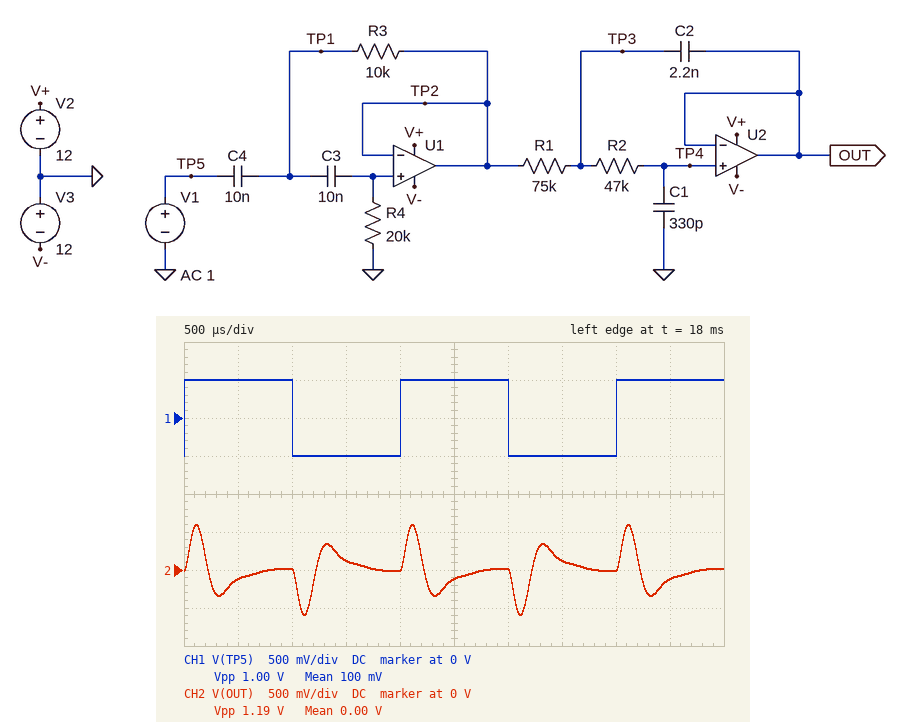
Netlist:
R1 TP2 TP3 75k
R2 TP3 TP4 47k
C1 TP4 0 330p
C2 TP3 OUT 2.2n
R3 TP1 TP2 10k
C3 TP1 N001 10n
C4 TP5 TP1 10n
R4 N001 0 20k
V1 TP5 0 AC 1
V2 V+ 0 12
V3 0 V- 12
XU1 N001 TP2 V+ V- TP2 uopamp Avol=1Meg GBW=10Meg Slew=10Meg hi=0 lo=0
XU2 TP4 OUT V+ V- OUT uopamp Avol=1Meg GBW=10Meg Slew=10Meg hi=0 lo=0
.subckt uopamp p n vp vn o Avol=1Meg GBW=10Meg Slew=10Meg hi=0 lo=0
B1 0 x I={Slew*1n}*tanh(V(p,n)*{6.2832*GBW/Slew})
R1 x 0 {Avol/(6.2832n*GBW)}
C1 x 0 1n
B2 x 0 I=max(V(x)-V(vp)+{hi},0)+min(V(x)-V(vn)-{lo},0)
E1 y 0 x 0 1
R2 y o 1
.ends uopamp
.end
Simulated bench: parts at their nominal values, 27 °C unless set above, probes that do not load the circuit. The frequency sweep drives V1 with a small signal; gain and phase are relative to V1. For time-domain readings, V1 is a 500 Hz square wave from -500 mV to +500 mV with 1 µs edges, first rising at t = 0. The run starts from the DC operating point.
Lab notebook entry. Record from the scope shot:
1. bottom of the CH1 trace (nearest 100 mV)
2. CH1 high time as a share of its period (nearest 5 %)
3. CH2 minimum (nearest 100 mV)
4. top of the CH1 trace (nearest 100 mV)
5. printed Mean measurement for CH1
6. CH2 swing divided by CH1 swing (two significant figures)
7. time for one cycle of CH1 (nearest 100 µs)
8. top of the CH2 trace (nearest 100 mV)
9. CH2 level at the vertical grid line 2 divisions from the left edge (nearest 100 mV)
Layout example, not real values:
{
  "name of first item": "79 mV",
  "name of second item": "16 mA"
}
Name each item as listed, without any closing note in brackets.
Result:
{
  "bottom of the CH1 trace": "-500 mV",
  "CH1 high time as a share of its period": "50 %",
  "CH2 minimum": "-600 mV",
  "top of the CH1 trace": "500 mV",
  "printed Mean measurement for CH1": "100 mV",
  "CH2 swing divided by CH1 swing": "1.2",
  "time for one cycle of CH1": "2.0 ms",
  "top of the CH2 trace": "600 mV",
  "CH2 level at the vertical grid line 2 divisions from the left edge": "0 V"
}
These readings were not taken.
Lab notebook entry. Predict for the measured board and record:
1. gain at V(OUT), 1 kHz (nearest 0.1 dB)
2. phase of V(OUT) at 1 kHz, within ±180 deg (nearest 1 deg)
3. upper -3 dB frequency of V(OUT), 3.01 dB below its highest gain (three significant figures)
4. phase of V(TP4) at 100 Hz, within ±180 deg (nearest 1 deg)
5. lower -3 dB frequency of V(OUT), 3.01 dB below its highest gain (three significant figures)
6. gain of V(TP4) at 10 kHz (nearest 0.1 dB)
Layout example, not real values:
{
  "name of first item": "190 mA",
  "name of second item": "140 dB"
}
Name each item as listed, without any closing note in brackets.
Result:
{
  "gain at V(OUT), 1 kHz": "-3.6 dB",
  "phase of V(OUT) at 1 kHz, within ±180 deg": "84 deg",
  "upper -3 dB frequency of V(OUT), 3.01 dB below its highest gain": "3.76 kHz",
  "phase of V(TP4) at 100 Hz, within ±180 deg": "171 deg",
  "lower -3 dB frequency of V(OUT), 3.01 dB below its highest gain": "1.39 kHz",
  "gain of V(TP4) at 10 kHz": "-19.5 dB"
}
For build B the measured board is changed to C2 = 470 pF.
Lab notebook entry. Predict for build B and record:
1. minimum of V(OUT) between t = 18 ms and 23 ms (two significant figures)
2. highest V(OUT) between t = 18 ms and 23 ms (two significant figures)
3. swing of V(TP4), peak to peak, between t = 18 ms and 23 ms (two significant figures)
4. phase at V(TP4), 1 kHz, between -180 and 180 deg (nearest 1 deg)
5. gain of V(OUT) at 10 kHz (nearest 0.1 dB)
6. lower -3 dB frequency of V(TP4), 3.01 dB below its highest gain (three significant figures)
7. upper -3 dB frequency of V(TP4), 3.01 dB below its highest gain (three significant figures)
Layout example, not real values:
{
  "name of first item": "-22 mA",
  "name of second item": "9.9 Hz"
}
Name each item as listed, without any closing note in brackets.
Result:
{
  "minimum of V(OUT) between t = 18 ms and 23 ms": "-580 mV",
  "highest V(OUT) between t = 18 ms and 23 ms": "580 mV",
  "swing of V(TP4), peak to peak, between t = 18 ms and 23 ms": "1.2 V",
  "phase at V(TP4), 1 kHz, between -180 and 180 deg": "85 deg",
  "gain of V(OUT) at 10 kHz": "-8.9 dB",
  "lower -3 dB frequency of V(TP4), 3.01 dB below its highest gain": "1.05 kHz",
  "upper -3 dB frequency of V(TP4), 3.01 dB below its highest gain": "6.03 kHz"
}
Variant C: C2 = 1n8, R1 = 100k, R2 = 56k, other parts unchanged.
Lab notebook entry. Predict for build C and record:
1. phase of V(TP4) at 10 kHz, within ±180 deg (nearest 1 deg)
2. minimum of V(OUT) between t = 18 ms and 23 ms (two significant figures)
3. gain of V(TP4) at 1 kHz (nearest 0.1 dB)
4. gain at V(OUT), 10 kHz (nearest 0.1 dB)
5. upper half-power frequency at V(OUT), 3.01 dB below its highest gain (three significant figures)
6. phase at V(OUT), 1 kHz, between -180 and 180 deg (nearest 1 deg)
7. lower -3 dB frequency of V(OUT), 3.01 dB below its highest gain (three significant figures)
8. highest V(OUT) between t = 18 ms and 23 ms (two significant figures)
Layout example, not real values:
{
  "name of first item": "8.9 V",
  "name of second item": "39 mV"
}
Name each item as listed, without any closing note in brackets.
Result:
{
  "phase of V(TP4) at 10 kHz, within ±180 deg": "-156 deg",
  "minimum of V(OUT) between t = 18 ms and 23 ms": "-520 mV",
  "gain of V(TP4) at 1 kHz": "-3.5 dB",
  "gain at V(OUT), 10 kHz": "-22.0 dB",
  "upper half-power frequency at V(OUT), 3.01 dB below its highest gain": "3.31 kHz",
  "phase at V(OUT), 1 kHz, between -180 and 180 deg": "79 deg",
  "lower -3 dB frequency of V(OUT), 3.01 dB below its highest gain": "1.23 kHz",
  "highest V(OUT) between t = 18 ms and 23 ms": "520 mV"
}
